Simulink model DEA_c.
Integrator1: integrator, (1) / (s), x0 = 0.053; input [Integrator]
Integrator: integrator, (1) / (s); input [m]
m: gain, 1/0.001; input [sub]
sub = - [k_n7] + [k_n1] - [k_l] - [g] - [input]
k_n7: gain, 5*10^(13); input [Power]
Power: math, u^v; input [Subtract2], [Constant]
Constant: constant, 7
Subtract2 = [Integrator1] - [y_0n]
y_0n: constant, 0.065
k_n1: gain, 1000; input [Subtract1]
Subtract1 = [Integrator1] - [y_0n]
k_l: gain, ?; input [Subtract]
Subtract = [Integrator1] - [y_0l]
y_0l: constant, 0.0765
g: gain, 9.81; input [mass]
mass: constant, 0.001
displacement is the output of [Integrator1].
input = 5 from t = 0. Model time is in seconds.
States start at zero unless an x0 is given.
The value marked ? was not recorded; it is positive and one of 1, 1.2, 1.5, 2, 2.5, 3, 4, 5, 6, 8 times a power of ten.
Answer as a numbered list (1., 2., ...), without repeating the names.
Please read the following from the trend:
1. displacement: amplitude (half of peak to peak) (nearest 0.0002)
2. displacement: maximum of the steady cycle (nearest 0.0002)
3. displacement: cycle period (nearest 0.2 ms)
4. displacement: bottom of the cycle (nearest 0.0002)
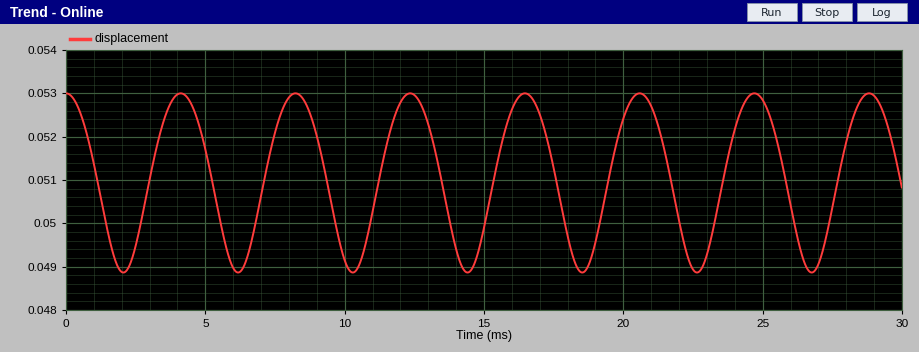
1. 0.0020
2. 0.0530
3. 4.2 ms
4. 0.0488
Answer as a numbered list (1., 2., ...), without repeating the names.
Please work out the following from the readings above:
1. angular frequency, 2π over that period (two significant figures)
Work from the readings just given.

1. 1.5 rad/ms
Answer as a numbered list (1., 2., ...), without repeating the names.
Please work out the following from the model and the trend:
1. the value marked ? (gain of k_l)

1. 500
